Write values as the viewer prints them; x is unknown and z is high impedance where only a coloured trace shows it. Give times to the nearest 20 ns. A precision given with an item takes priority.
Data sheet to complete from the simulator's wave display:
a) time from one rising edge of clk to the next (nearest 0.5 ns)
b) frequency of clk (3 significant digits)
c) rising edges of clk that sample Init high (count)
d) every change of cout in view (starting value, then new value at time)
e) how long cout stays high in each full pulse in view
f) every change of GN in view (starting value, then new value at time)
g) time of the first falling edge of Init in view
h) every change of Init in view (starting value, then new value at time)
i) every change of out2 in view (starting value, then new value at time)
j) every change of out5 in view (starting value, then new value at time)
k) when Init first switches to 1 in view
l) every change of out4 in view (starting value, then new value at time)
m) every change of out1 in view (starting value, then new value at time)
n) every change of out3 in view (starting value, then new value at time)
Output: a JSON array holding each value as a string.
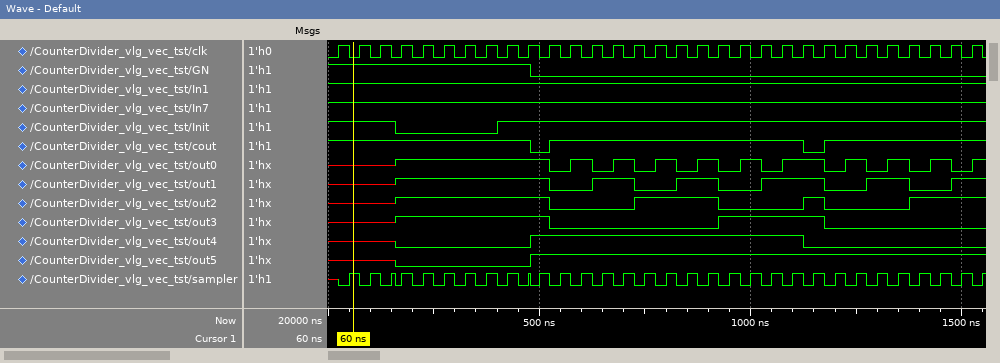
["50 ns", "20.0 MHz", "26", "1, 0 at 480 ns, 1 at 520 ns, 0 at 1120 ns, 1 at 1180 ns", "600 ns", "1, 0 at 480 ns", "160 ns", "1, 0 at 160 ns, 1 at 400 ns", "x, 1 at 160 ns, 0 at 520 ns, 1 at 720 ns, 0 at 920 ns, 1 at 1120 ns, 0 at 1180 ns, 1 at 1380 ns", "x, 0 at 160 ns, 1 at 480 ns", "400 ns", "x, 0 at 160 ns, 1 at 480 ns, 0 at 1120 ns", "x, 1 at 160 ns, 0 at 520 ns, 1 at 620 ns, 0 at 720 ns, 1 at 820 ns, 0 at 920 ns, 1 at 1020 ns, 0 at 1180 ns, 1 at 1280 ns, 0 at 1380 ns, 1 at 1480 ns", "x, 1 at 160 ns, 0 at 520 ns, 1 at 920 ns, 0 at 1180 ns"]
